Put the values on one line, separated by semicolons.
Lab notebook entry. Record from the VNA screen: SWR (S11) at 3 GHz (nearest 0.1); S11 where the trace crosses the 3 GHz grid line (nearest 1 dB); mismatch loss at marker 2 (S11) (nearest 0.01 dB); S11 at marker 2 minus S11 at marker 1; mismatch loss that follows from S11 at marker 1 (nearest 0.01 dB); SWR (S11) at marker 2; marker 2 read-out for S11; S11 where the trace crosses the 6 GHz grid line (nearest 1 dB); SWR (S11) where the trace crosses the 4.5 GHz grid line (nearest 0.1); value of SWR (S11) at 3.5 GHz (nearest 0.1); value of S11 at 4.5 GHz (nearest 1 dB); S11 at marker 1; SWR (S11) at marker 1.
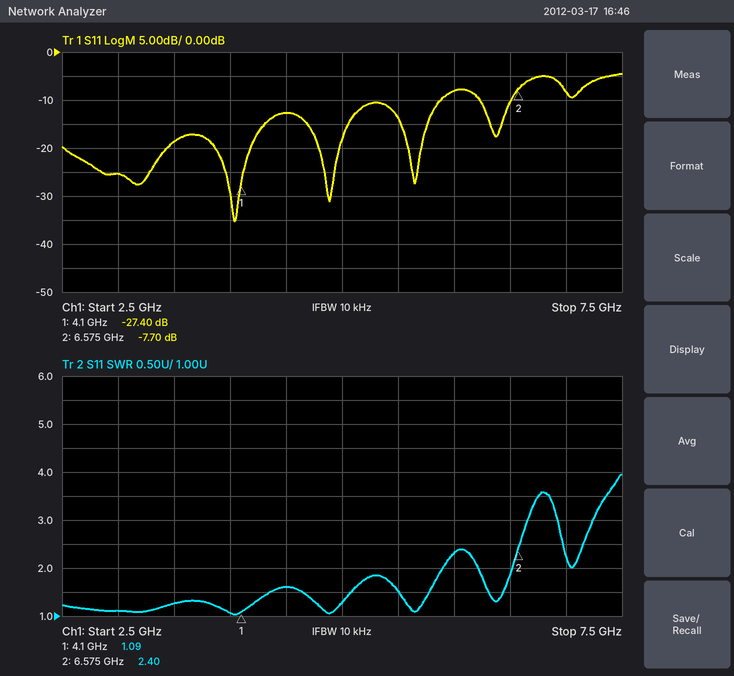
1.1; -25 dB; 0.81 dB; 19.70 dB; 0.01 dB; 2.40; -7.70 dB; -8 dB; 1.6; 1.3; -13 dB; -27.40 dB; 1.09
